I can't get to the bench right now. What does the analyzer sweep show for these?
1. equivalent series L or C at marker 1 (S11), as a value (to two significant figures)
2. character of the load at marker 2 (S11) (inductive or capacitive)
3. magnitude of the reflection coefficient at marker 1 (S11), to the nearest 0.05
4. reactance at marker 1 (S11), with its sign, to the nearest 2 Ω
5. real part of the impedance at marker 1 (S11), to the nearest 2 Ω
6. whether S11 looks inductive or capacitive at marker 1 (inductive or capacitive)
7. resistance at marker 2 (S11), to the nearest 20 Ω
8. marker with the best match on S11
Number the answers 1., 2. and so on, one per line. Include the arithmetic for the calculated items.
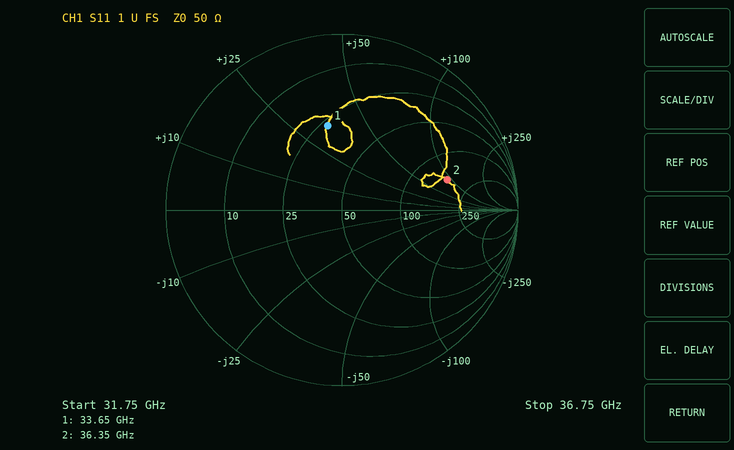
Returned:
1. L = 34 Ω/(2π × 33.65 GHz) ≈ 161 pH, so 160 pH to two significant figures
2. inductive
3. 0.50
4. +34 Ω
5. 28 Ω
6. inductive
7. 160 Ω
8. marker 1
